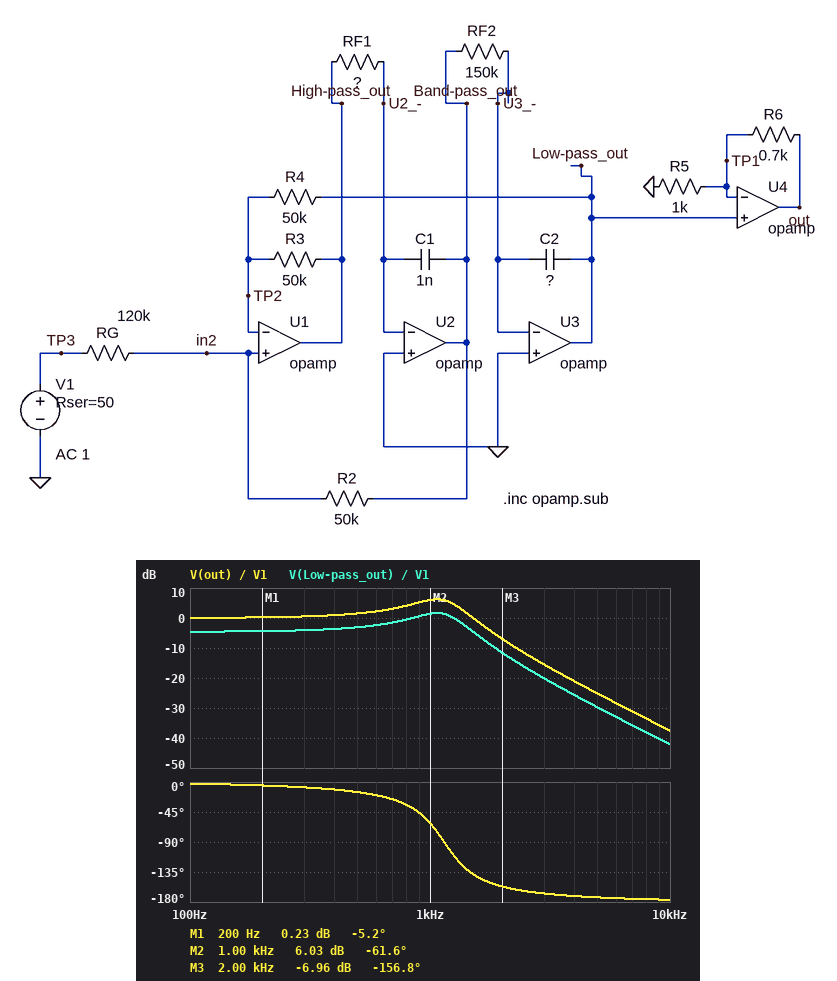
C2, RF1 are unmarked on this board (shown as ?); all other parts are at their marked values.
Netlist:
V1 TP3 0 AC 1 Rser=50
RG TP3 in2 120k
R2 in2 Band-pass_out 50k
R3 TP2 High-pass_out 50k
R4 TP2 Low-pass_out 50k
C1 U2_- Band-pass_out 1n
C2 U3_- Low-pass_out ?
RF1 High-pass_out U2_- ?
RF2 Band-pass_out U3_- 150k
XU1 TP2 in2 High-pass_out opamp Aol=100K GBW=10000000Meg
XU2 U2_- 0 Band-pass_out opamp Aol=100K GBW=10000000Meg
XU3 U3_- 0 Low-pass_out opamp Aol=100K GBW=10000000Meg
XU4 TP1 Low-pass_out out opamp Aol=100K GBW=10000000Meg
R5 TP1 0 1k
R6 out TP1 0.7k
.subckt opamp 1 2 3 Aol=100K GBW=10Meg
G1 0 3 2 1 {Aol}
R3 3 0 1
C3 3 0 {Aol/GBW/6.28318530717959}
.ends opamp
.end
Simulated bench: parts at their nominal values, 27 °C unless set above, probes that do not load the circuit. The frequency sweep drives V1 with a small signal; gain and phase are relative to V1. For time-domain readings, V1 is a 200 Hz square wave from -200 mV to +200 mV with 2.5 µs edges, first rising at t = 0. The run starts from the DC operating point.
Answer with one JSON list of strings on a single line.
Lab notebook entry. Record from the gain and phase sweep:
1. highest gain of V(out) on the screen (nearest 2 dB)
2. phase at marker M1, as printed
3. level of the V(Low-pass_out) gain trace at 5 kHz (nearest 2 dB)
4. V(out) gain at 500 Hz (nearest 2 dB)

["6 dB", "-5.2 deg", "-30 dB", "2 dB"]
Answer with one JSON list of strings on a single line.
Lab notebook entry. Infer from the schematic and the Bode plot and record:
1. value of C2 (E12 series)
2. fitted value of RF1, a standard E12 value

["330 pF", "390 kΩ"]
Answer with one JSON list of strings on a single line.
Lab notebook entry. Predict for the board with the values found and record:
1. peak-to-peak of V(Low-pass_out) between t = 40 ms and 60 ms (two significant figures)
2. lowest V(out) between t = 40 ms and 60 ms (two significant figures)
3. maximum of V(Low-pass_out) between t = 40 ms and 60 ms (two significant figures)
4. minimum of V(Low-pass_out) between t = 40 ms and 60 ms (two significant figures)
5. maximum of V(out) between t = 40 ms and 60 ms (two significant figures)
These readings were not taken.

["440 mV", "-380 mV", "220 mV", "-220 mV", "380 mV"]
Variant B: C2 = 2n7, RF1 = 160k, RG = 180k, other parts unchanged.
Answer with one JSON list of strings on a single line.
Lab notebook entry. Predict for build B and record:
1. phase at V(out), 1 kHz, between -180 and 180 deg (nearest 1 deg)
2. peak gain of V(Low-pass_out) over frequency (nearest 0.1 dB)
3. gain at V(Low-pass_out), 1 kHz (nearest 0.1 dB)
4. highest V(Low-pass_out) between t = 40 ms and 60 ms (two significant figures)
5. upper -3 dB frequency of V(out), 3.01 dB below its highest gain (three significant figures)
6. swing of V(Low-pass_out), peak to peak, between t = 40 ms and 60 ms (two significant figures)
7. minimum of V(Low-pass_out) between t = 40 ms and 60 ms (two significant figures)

["-111 deg", "-7.2 dB", "-19.9 dB", "85 mV", "297 Hz", "170 mV", "-85 mV"]
